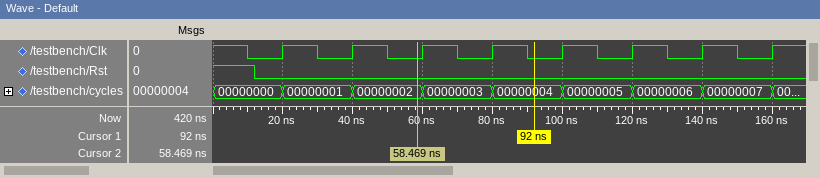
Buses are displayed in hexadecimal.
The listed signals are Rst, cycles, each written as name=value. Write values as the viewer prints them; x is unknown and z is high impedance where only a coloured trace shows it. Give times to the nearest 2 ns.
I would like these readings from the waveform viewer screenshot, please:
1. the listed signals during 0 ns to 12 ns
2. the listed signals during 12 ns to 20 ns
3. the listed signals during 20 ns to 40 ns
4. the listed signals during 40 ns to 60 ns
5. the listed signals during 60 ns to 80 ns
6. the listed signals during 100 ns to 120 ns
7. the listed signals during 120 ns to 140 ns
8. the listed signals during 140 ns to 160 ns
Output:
Rst=1, cycles=00000000
Rst=0, cycles=00000000
Rst=0, cycles=00000001
Rst=0, cycles=00000002
Rst=0, cycles=00000003
Rst=0, cycles=00000005
Rst=0, cycles=00000006
Rst=0, cycles=00000007
